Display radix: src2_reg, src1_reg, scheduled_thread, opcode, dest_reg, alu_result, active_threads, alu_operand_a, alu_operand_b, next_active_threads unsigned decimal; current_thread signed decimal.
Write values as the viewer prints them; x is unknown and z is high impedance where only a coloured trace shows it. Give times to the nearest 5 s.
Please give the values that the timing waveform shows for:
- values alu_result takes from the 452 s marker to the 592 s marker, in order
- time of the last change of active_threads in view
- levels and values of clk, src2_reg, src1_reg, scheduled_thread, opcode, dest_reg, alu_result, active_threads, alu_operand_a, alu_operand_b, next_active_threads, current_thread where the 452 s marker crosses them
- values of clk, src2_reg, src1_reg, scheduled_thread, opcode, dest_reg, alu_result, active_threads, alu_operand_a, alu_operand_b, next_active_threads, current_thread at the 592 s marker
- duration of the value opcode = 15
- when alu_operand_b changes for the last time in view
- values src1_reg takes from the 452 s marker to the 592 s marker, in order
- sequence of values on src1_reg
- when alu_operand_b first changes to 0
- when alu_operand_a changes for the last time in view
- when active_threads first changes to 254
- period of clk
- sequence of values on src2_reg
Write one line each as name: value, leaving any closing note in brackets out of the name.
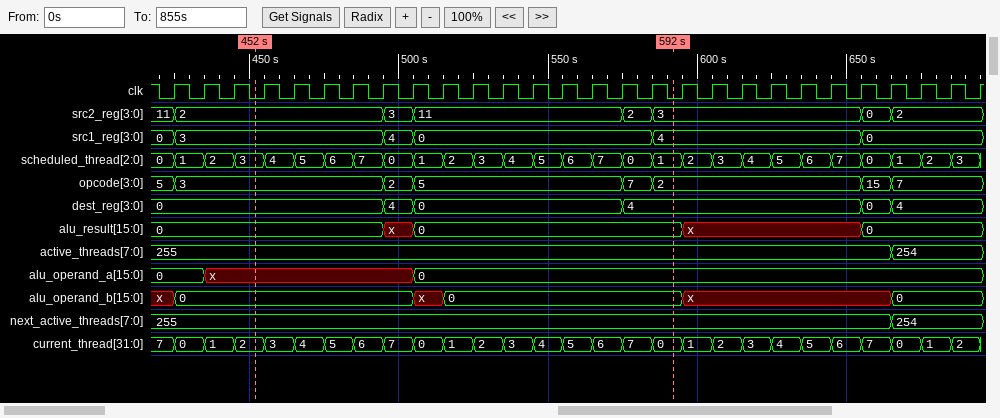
values alu_result takes from the 452 s marker to the 592 s marker, in order: 0, x, 0
time of the last change of active_threads in view: 665 s
levels and values of clk, src2_reg, src1_reg, scheduled_thread, opcode, dest_reg, alu_result, active_threads, alu_operand_a, alu_operand_b, next_active_threads, current_thread where the 452 s marker crosses them: clk=0, src2_reg=2, src1_reg=3, scheduled_thread=3, opcode=3, dest_reg=0, alu_result=0, active_threads=255, alu_operand_a=x, alu_operand_b=0, next_active_threads=255, current_thread=2
values of clk, src2_reg, src1_reg, scheduled_thread, opcode, dest_reg, alu_result, active_threads, alu_operand_a, alu_operand_b, next_active_threads, current_thread at the 592 s marker: clk=0, src2_reg=3, src1_reg=4, scheduled_thread=1, opcode=2, dest_reg=4, alu_result=0, active_threads=255, alu_operand_a=0, alu_operand_b=0, next_active_threads=255, current_thread=0
duration of the value opcode = 15: 10 s
when alu_operand_b changes for the last time in view: 665 s
values src1_reg takes from the 452 s marker to the 592 s marker, in order: 3, 4, 0, 4
sequence of values on src1_reg: 0, 3, 4, 0, 4, 0
when alu_operand_b first changes to 0: 425 s
when alu_operand_a changes for the last time in view: 505 s
when active_threads first changes to 254: 665 s
period of clk: 10 s
sequence of values on src2_reg: 11, 2, 3, 11, 2, 3, 0, 2
